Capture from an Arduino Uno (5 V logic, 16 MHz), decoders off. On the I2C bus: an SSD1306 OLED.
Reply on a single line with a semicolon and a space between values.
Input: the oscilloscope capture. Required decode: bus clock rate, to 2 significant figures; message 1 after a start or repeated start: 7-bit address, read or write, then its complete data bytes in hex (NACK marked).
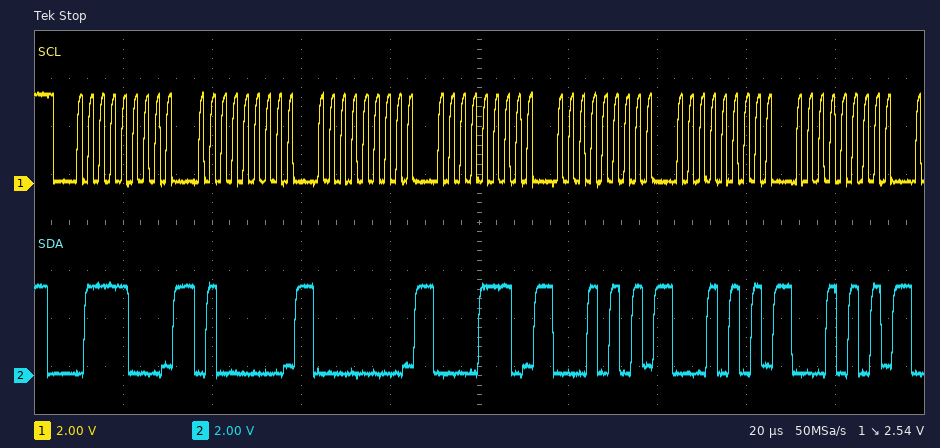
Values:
400 kHz; 0x3C write: 40 00 0E 15 15 15
